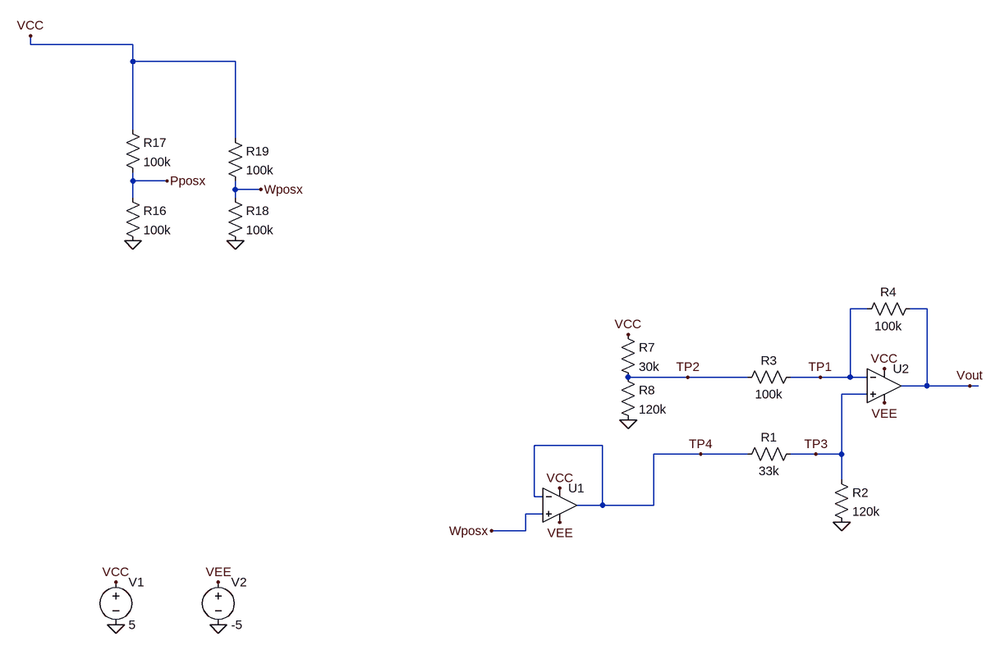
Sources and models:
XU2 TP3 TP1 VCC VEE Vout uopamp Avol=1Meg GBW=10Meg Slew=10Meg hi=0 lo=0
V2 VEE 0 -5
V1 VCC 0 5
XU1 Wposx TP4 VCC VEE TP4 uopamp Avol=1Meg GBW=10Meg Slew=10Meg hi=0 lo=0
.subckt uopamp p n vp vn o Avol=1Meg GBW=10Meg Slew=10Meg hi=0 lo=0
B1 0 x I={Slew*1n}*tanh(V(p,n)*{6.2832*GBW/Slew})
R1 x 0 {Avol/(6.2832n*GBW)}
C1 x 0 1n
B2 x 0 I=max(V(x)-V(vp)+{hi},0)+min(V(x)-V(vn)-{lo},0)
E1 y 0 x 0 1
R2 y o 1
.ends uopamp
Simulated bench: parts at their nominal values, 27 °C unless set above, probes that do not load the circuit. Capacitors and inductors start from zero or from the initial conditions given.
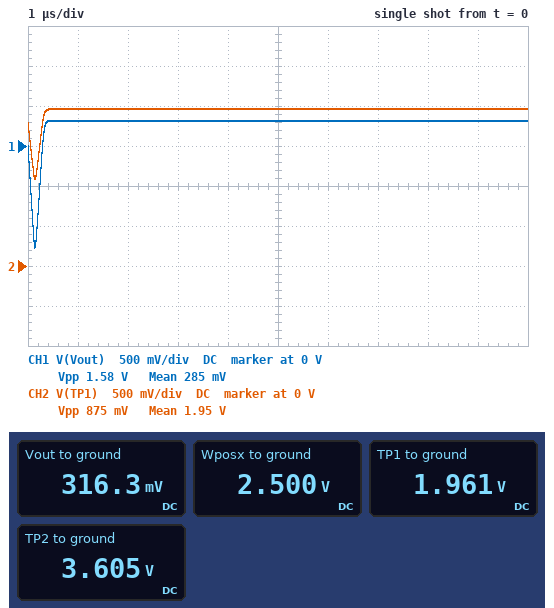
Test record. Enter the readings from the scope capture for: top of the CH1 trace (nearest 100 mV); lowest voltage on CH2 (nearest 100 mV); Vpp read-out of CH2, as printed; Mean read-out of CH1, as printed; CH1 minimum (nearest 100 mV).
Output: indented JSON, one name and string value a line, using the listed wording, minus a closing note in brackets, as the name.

{
  "top of the CH1 trace": "300 mV",
  "lowest voltage on CH2": "1.1 V",
  "Vpp read-out of CH2, as printed": "875 mV",
  "Mean read-out of CH1, as printed": "285 mV",
  "CH1 minimum": "-1.3 V"
}
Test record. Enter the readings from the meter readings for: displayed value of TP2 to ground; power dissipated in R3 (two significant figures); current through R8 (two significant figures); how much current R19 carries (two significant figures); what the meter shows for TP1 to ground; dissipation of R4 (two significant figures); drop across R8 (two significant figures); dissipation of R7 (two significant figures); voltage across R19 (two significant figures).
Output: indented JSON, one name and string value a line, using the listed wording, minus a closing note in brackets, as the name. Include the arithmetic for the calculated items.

{
  "displayed value of TP2 to ground": "3.605 V",
  "power dissipated in R3": "(3.605 V - 1.961 V)^2 / 100 kΩ = 27 µW",
  "current through R8": "(3.605 V) / 120 kΩ = 30 µA",
  "how much current R19 carries": "(5 V - 2.5 V) / 100 kΩ = 25 µA",
  "what the meter shows for TP1 to ground": "1.961 V",
  "dissipation of R4": "(1.961 V - 316.3 mV)^2 / 100 kΩ = 27 µW",
  "drop across R8": "3.605 V = 3.6 V",
  "dissipation of R7": "(5 V - 3.605 V)^2 / 30 kΩ = 65 µW",
  "voltage across R19": "5 V - 2.5 V = 2.5 V"
}
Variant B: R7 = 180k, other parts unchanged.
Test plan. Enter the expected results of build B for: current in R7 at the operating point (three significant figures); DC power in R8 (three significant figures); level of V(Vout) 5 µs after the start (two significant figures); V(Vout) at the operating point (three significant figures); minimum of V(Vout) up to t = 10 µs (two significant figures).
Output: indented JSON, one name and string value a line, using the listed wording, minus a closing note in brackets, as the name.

{
  "current in R7 at the operating point": "16.8 µA",
  "DC power in R8": "32.8 µW",
  "level of V(Vout) 5 µs after the start": "1.9 V",
  "V(Vout) at the operating point": "1.94 V",
  "minimum of V(Vout) up to t = 10 µs": "-460 mV"
}
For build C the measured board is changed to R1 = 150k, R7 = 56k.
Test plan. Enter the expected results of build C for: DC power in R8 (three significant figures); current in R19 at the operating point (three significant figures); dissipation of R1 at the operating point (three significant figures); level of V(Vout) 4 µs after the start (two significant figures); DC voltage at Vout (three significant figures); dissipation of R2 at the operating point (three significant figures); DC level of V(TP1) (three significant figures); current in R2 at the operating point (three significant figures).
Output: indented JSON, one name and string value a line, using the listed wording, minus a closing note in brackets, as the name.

{
  "DC power in R8": "64.1 µW",
  "current in R19 at the operating point": "25.0 µA",
  "dissipation of R1 at the operating point": "12.9 µW",
  "level of V(Vout) 4 µs after the start": "-550 mV",
  "DC voltage at Vout": "-552 mV",
  "dissipation of R2 at the operating point": "10.3 µW",
  "DC level of V(TP1)": "1.11 V",
  "current in R2 at the operating point": "9.26 µA"
}
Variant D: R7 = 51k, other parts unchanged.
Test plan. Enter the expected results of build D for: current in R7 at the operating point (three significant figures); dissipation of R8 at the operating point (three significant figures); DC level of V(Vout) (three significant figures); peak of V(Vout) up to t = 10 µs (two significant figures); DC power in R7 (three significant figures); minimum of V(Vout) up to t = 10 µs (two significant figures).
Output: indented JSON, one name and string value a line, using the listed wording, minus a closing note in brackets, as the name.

{
  "current in R7 at the operating point": "37.2 µA",
  "dissipation of R8 at the operating point": "80.1 µW",
  "DC level of V(Vout)": "821 mV",
  "peak of V(Vout) up to t = 10 µs": "820 mV",
  "DC power in R7": "70.7 µW",
  "minimum of V(Vout) up to t = 10 µs": "-1.0 V"
}
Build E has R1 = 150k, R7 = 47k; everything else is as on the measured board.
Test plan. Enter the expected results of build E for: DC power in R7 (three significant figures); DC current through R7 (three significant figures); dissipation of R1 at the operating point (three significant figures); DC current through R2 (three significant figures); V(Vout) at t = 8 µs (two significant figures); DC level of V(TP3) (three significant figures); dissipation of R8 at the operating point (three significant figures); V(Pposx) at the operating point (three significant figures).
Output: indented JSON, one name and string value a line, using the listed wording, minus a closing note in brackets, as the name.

{
  "DC power in R7": "88.0 µW",
  "DC current through R7": "43.3 µA",
  "dissipation of R1 at the operating point": "12.9 µW",
  "DC current through R2": "9.26 µA",
  "V(Vout) at t = 8 µs": "-740 mV",
  "DC level of V(TP3)": "1.11 V",
  "dissipation of R8 at the operating point": "73.3 µW",
  "V(Pposx) at the operating point": "2.50 V"
}
